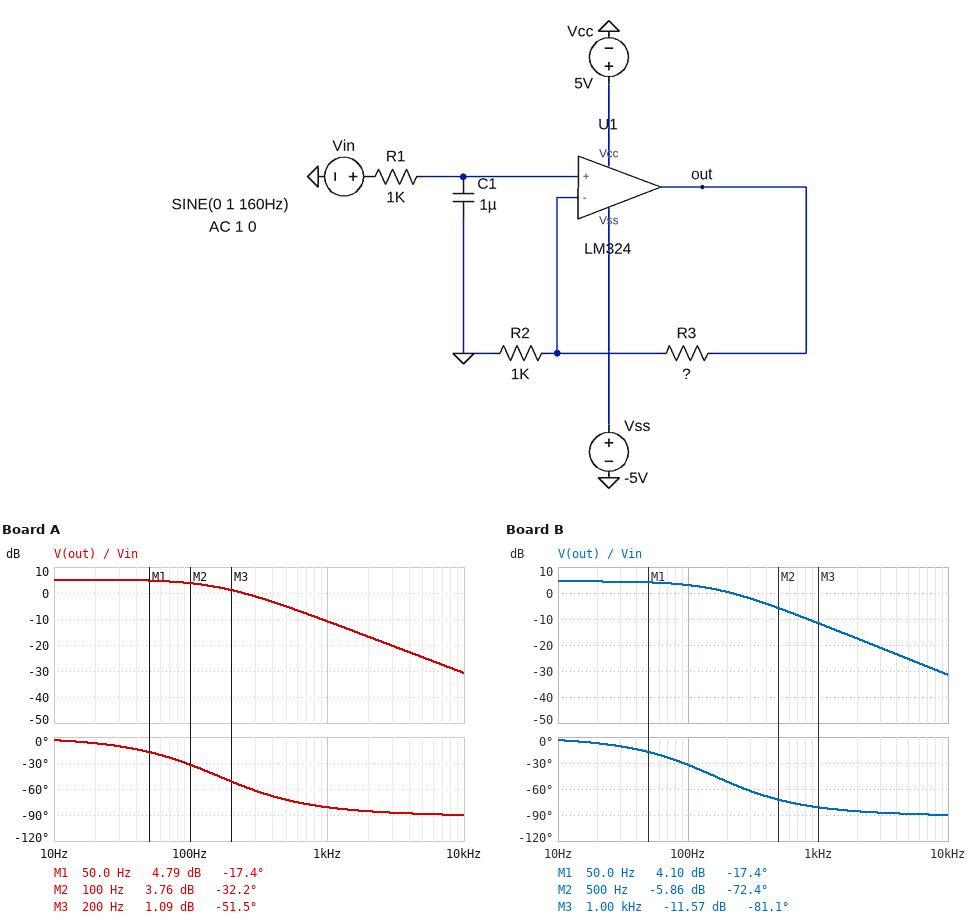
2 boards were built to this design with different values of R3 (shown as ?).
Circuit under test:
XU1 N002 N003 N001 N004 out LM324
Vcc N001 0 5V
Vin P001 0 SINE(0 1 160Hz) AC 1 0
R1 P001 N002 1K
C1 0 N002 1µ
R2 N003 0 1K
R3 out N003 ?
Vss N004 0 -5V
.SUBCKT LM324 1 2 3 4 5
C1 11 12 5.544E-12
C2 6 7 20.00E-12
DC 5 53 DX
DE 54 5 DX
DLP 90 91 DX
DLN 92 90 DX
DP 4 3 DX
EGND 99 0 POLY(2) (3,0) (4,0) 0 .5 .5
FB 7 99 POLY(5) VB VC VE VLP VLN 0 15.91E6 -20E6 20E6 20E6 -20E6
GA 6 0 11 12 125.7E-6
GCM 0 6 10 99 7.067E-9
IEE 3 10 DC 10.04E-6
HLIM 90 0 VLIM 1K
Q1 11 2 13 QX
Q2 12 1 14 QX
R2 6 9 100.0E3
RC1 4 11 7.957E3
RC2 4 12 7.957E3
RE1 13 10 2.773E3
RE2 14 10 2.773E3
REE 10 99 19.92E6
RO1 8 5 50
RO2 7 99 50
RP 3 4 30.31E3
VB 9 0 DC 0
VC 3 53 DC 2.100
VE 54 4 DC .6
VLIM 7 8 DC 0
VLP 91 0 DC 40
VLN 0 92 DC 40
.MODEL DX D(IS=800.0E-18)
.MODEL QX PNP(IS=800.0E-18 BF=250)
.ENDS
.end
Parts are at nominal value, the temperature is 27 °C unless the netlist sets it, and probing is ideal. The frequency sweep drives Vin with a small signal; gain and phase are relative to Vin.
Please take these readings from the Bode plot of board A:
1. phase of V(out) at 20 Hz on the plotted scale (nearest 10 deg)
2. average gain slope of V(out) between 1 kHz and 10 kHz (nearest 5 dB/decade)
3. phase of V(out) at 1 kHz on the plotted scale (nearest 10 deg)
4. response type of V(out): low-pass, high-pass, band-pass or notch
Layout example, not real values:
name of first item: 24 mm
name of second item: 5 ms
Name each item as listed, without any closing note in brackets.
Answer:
phase of V(out) at 20 Hz on the plotted scale: -10 deg
average gain slope of V(out) between 1 kHz and 10 kHz: -20 dB/decade
phase of V(out) at 1 kHz on the plotted scale: -80 deg
response type of V(out): low-pass, high-pass, band-pass or notch: low-pass
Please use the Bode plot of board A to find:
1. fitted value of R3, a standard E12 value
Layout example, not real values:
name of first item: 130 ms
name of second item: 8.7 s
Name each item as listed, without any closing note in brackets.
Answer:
fitted value of R3, a standard E12 value: 820 Ω
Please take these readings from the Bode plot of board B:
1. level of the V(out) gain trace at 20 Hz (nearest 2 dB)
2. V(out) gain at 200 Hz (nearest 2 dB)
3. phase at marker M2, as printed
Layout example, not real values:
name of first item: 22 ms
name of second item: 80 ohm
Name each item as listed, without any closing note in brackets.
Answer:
level of the V(out) gain trace at 20 Hz: 4 dB
V(out) gain at 200 Hz: 0 dB
phase at marker M2, as printed: -72.4 deg
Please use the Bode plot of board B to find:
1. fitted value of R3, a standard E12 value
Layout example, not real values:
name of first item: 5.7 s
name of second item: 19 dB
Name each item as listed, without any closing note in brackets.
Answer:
fitted value of R3, a standard E12 value: 680 Ω
